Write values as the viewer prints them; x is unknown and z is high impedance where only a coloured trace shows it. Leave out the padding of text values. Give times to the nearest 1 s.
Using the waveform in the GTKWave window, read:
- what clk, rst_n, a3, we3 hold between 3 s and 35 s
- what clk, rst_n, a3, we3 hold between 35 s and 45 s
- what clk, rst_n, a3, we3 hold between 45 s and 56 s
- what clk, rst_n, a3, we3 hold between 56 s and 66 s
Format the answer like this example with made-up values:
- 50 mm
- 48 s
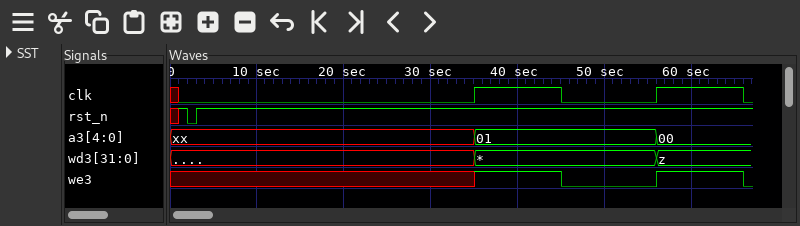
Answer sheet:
- clk=0, rst_n=1, a3=xx, we3=x
- clk=1, rst_n=1, a3=01, we3=1
- clk=0, rst_n=1, a3=01, we3=0
- clk=1, rst_n=1, a3=00, we3=1
